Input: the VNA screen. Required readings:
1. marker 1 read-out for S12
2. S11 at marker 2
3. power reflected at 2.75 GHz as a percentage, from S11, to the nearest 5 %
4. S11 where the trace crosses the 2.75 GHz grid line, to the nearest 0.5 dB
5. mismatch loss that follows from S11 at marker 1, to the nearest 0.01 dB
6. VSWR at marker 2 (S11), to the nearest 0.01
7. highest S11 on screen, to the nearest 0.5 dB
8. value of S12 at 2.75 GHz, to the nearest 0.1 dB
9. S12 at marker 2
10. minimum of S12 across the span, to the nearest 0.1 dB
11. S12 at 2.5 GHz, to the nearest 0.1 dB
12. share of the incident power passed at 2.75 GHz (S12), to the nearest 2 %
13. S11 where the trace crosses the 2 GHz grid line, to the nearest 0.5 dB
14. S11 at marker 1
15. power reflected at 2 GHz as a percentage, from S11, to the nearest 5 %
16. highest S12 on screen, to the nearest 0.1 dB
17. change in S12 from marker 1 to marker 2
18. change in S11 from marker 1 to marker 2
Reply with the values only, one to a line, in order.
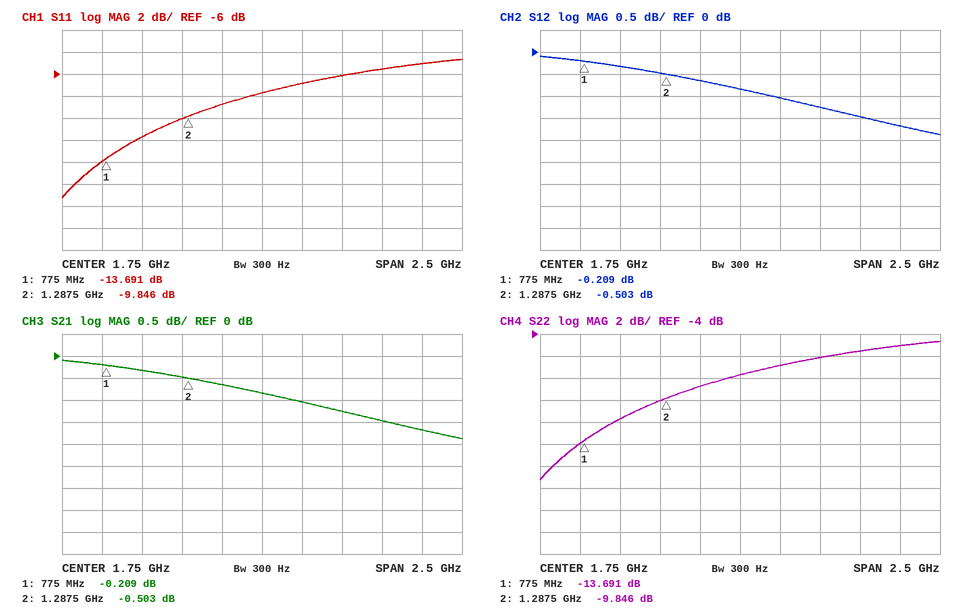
-0.209 dB
-9.846 dB
30 %
-5.0 dB
0.19 dB
1.95
-4.5 dB
-1.7 dB
-0.503 dB
-1.9 dB
-1.5 dB
68 %
-7.0 dB
-13.691 dB
20 %
-0.1 dB
-0.294 dB
3.845 dB
